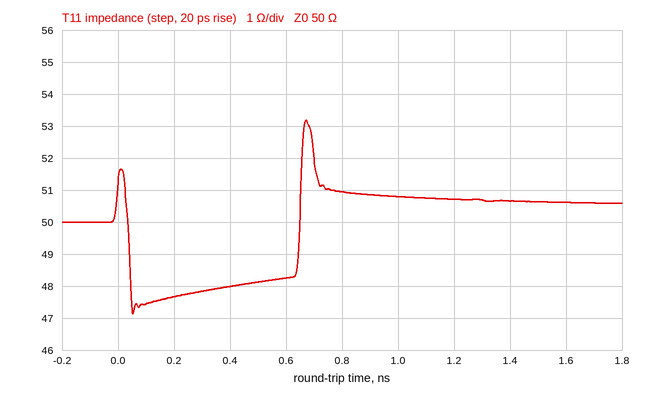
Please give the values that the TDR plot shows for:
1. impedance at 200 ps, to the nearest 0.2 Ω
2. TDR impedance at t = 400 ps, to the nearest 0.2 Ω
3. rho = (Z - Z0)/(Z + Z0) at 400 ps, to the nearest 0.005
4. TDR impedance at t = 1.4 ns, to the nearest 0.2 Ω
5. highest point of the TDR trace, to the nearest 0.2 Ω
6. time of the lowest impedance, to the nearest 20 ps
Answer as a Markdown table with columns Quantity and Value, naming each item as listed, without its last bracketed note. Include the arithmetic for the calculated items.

| Quantity | Value |
|---|---|
| impedance at 200 ps, to the nearest 0.2 Ω | 47.6 Ω |
| TDR impedance at t = 400 ps, to the nearest 0.2 Ω | 48.0 Ω |
| rho = (Z - Z0)/(Z + Z0) at 400 ps, to the nearest 0.005 | (48 − 50)/(48 + 50) ≈ -0.020 |
| TDR impedance at t = 1.4 ns, to the nearest 0.2 Ω | 50.6 Ω |
| highest point of the TDR trace, to the nearest 0.2 Ω | 53.2 Ω |
| time of the lowest impedance, to the nearest 20 ps | 60 ps |
